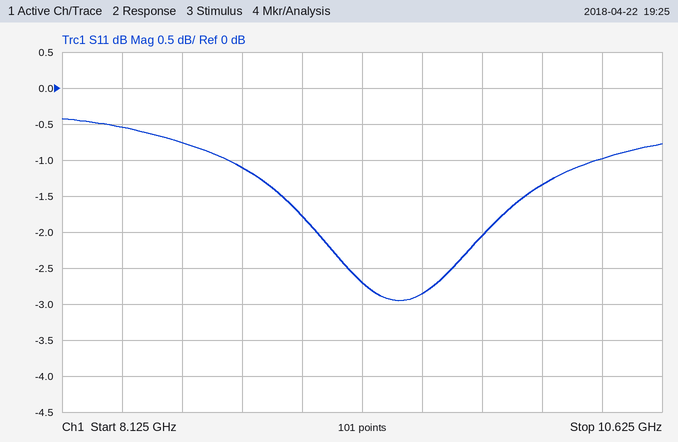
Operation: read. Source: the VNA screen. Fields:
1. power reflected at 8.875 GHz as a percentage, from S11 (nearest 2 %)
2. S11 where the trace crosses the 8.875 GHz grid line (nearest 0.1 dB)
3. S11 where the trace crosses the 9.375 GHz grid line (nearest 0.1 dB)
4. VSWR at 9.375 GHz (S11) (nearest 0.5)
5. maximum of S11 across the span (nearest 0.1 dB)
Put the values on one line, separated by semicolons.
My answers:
78 %; -1.1 dB; -2.7 dB; 6.5; -0.4 dB
